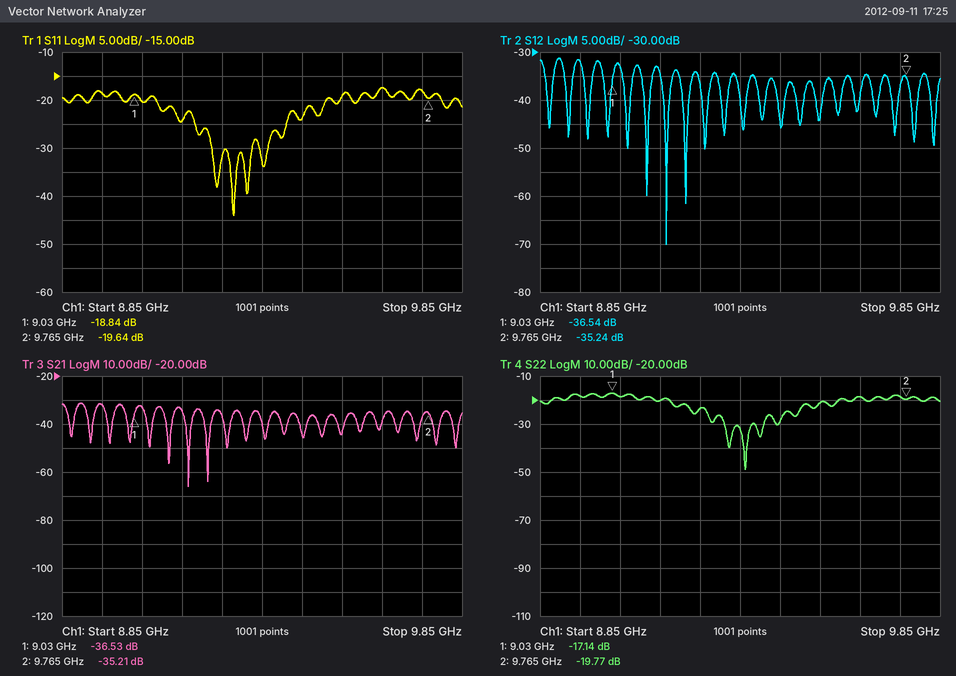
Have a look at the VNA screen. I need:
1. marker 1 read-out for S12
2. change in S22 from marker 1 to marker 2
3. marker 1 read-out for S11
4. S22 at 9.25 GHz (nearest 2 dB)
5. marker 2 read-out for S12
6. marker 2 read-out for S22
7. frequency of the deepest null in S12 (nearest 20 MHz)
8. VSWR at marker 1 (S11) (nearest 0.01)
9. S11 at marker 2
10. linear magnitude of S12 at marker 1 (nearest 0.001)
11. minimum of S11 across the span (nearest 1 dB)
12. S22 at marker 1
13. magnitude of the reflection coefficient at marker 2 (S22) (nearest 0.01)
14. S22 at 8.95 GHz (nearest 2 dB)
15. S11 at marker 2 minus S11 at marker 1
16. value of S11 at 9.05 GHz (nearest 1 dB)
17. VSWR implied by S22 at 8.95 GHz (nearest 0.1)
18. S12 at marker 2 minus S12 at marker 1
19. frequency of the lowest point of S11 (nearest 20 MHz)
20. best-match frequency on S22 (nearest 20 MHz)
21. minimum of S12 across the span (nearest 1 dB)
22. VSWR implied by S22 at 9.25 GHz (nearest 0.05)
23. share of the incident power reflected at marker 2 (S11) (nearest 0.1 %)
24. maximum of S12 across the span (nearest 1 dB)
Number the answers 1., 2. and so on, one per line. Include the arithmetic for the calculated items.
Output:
1. -36.54 dB
2. -19.77 − (-17.14) = -2.63 dB
3. -18.84 dB
4. -24 dB
5. -35.24 dB
6. -19.77 dB
7. 9.16 GHz
8. (1 + 0.1143)/(1 − 0.1143) ≈ 1.26
9. -19.64 dB
10. 10^(-36.54/20) ≈ 0.015
11. -44 dB
12. -17.14 dB
13. 10^(-19.77/20) ≈ 0.10
14. -18 dB
15. -19.64 − (-18.84) = -0.80 dB
16. -20 dB
17. |Γ| = 10^(-18/20) = 0.1259; VSWR = (1 + 0.1259)/(1 − 0.1259) ≈ 1.3
18. -35.24 − (-36.54) = 1.30 dB
19. 9.28 GHz
20. 9.36 GHz
21. -70 dB
22. |Γ| = 10^(-24/20) = 0.0631; VSWR = (1 + 0.0631)/(1 − 0.0631) ≈ 1.13, so 1.15 to the nearest 0.05
23. 10^(-19.64/10) ≈ 1.1 %
24. -31 dB
